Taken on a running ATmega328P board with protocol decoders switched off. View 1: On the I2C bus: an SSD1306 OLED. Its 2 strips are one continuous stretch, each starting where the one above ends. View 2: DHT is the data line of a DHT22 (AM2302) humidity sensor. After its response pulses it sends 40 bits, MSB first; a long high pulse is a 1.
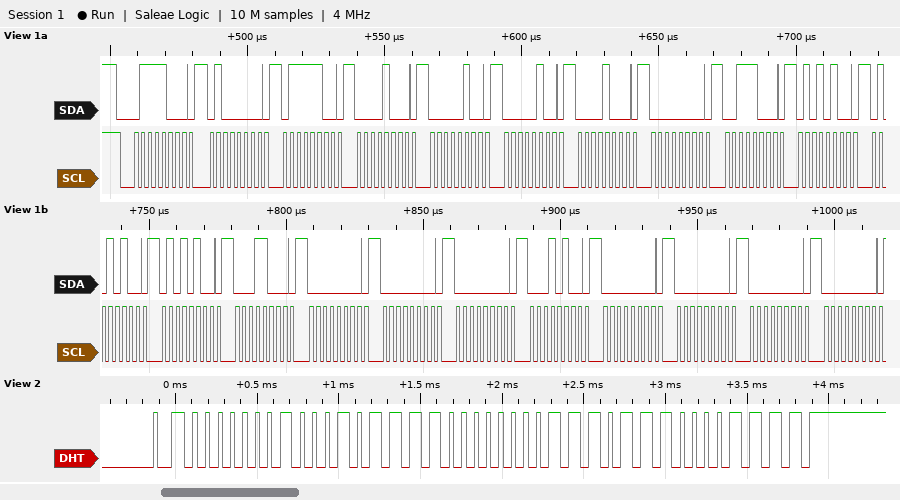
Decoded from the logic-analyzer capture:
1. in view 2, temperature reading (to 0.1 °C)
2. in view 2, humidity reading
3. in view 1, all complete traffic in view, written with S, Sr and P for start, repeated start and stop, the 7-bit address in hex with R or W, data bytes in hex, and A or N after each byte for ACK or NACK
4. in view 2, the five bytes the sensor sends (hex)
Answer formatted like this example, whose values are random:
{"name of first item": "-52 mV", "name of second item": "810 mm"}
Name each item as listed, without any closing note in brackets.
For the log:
{"in view 2, temperature reading": "-11.9 °C", "in view 2, humidity reading": "27.9 %", "in view 1, all complete traffic in view, written with S, Sr and P for start, repeated start and stop, the 7-bit address in hex with R or W, data bytes in hex, and A or N after each byte for ACK or NACK": "S 3CW A 40 A 7C A 08 A 04 A 04 A 08 A 00 A 38 A 54 A 54 A 54 A 18 A 00 A 00 A 00 A 14 A 00 A 00 A 00 A 00 A", "in view 2, the five bytes the sensor sends": "01 17 80 77 0F"}
